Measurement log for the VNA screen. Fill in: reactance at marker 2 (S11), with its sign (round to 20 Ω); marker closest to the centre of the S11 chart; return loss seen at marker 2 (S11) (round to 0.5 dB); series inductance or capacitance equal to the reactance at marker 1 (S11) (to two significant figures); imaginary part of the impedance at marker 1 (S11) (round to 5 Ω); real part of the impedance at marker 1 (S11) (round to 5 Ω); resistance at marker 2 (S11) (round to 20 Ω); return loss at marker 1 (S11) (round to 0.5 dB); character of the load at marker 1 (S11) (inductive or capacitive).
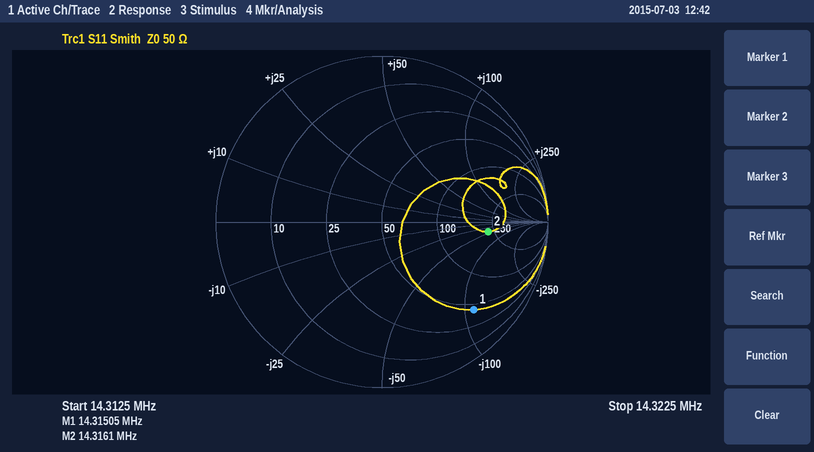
-40 Ω
marker 2
4.0 dB
100 pF
-110 Ω
45 Ω
220 Ω
2.5 dB
capacitive
